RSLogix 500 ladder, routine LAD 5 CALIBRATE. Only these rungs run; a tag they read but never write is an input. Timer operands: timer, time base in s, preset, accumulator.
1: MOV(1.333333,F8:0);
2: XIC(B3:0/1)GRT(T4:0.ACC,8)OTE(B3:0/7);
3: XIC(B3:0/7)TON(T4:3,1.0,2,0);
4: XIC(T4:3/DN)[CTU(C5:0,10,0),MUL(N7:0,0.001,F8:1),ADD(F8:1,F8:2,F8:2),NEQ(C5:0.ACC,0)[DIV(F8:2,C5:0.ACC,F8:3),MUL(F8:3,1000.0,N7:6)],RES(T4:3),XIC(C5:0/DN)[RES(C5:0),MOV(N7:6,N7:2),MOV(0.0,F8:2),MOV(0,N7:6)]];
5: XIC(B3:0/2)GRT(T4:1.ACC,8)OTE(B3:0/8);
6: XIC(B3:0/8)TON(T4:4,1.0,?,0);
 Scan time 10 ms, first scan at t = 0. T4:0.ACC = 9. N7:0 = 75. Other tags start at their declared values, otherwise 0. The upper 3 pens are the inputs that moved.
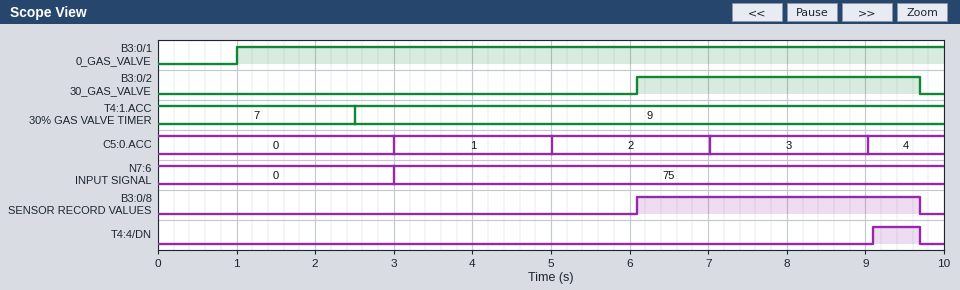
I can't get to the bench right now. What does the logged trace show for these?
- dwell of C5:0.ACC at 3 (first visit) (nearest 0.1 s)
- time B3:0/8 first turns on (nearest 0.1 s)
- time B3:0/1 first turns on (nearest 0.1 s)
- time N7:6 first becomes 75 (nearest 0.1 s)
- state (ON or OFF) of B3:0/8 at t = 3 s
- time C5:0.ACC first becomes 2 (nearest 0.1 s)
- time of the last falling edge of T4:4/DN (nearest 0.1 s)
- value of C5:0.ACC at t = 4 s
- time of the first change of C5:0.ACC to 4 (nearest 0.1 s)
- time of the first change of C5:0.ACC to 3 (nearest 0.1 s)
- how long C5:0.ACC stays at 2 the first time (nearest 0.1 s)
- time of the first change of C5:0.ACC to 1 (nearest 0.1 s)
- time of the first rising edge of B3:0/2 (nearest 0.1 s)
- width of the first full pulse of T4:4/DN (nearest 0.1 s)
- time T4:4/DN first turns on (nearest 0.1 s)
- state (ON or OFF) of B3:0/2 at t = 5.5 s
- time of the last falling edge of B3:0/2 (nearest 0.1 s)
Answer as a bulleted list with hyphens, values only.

- 2.0 s
- 6.1 s
- 1.0 s
- 3.0 s
- OFF
- 5.0 s
- 9.7 s
- 1
- 9.0 s
- 7.0 s
- 2.0 s
- 3.0 s
- 6.1 s
- 0.6 s
- 9.1 s
- OFF
- 9.7 s
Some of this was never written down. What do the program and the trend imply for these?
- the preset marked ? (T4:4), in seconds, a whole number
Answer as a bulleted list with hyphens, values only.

- 3 s
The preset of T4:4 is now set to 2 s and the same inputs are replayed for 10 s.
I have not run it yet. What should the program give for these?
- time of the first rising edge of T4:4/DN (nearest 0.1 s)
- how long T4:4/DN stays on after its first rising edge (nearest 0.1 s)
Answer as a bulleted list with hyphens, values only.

- 8.1 s
- 1.6 s
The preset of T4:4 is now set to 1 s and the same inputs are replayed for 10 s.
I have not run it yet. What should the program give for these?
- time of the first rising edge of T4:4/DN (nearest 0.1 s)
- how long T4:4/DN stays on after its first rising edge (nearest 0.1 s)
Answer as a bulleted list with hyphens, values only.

- 7.1 s
- 2.6 s
